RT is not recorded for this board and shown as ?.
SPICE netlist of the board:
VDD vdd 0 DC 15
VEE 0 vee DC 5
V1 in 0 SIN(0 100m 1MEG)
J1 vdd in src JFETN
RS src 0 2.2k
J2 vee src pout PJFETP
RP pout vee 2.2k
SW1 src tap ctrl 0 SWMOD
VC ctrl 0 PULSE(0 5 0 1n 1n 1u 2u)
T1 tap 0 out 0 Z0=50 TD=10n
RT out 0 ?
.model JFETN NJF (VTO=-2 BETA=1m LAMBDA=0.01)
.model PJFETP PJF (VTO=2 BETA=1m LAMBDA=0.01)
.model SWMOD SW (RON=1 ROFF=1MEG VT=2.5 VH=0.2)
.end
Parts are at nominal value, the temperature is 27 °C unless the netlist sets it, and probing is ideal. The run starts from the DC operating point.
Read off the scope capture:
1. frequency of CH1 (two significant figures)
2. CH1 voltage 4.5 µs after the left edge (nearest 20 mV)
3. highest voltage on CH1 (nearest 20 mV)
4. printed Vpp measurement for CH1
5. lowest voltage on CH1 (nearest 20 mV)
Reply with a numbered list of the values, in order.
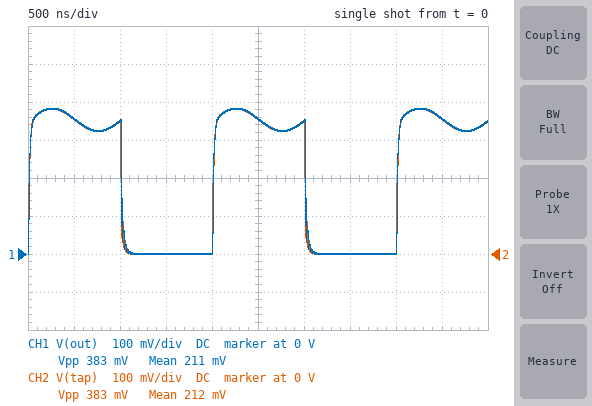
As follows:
1. 500 kHz
2. 360 mV
3. 380 mV
4. 383 mV
5. 0 V
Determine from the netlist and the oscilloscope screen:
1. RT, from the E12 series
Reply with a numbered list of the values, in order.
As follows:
1. 120 Ω
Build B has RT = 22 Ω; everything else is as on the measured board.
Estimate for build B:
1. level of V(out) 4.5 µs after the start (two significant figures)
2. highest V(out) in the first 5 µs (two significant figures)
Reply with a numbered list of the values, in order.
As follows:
1. 91 mV
2. 110 mV
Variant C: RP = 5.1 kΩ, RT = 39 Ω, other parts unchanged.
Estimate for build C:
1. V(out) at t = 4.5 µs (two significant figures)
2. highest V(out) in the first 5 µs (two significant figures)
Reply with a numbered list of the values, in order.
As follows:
1. 150 mV
2. 160 mV
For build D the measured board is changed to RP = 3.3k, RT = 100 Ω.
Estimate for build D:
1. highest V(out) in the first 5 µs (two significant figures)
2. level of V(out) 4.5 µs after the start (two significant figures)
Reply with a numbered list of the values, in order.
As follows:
1. 340 mV
2. 310 mV
